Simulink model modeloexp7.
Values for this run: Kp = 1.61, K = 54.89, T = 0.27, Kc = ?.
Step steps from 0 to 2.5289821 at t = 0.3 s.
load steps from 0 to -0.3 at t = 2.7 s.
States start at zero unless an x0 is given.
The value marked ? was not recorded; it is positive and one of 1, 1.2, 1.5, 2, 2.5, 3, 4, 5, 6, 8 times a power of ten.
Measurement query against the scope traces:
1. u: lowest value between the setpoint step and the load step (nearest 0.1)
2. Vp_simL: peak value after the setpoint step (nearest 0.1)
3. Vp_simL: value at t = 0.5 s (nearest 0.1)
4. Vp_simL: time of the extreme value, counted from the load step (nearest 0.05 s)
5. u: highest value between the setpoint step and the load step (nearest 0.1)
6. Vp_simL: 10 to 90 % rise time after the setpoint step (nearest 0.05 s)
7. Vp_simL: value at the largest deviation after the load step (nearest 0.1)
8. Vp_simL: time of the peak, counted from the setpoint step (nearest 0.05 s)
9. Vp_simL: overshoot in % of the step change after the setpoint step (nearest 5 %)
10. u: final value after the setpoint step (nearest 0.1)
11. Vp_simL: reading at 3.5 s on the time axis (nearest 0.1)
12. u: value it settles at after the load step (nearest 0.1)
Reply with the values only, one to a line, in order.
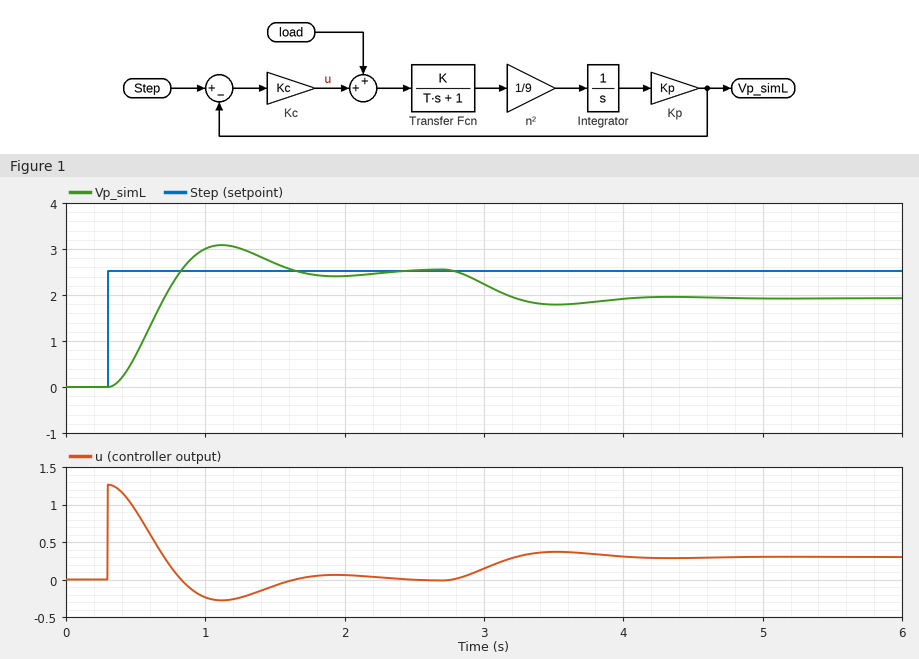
-0.3
3.1
0.7
0.80 s
1.3
0.35 s
1.8
0.80 s
20 %
0.0
1.8
0.3
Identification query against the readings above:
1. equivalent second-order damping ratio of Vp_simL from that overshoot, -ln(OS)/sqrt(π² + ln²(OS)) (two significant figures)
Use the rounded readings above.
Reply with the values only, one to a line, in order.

0.46
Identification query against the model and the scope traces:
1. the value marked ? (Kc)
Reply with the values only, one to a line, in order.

0.5
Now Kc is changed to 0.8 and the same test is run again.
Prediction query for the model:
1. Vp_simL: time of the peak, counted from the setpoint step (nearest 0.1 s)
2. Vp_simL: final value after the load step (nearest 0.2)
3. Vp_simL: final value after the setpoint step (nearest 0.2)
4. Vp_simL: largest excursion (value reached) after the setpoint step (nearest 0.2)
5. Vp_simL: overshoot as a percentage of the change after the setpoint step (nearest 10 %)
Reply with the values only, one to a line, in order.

0.6 s
2.2
2.6
3.4
30 %
